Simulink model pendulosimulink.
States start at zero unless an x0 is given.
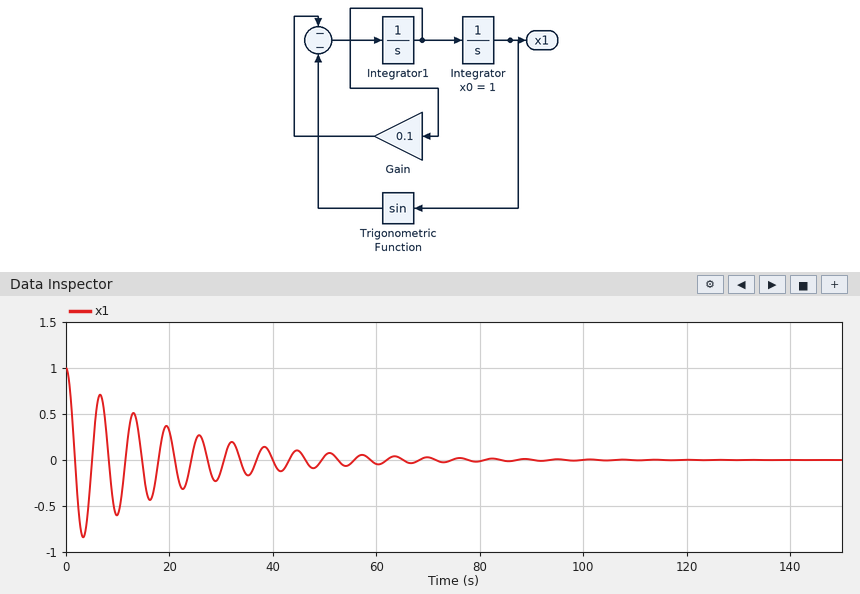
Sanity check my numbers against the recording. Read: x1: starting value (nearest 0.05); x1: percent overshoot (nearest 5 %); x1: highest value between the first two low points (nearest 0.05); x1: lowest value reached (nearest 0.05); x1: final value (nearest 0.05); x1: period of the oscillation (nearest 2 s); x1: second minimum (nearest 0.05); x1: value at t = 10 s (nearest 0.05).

1.00
85 %
0.70
-0.85
0.00
6 s
-0.60
-0.60
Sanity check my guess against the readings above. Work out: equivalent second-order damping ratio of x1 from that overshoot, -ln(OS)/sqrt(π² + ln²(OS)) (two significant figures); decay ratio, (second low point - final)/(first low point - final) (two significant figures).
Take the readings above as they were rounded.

0.052
0.71
